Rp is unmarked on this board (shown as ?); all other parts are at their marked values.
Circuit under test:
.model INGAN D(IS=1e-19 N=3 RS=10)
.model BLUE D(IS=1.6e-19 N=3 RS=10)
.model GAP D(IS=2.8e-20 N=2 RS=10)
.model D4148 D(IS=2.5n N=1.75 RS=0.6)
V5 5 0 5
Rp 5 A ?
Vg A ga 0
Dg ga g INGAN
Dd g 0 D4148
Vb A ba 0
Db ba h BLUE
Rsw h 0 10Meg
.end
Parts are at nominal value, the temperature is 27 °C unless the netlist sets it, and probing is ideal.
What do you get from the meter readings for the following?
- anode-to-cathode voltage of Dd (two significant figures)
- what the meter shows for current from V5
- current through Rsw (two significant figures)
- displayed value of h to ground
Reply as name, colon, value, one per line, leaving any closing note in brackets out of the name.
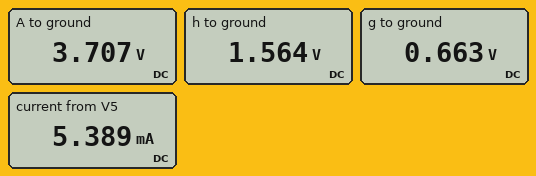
anode-to-cathode voltage of Dd: 660 mV
what the meter shows for current from V5: 5.389 mA
current through Rsw: 160 nA
displayed value of h to ground: 1.564 V
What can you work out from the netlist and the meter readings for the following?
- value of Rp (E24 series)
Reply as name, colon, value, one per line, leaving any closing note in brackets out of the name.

value of Rp: 240 Ω
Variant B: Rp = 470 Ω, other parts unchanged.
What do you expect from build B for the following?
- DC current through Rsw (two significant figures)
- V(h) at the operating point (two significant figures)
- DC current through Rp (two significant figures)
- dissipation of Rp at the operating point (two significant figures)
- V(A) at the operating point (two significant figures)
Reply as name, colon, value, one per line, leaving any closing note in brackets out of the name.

DC current through Rsw: 150 nA
V(h) at the operating point: 1.5 V
DC current through Rp: 3.0 mA
dissipation of Rp at the operating point: 4.1 mW
V(A) at the operating point: 3.6 V
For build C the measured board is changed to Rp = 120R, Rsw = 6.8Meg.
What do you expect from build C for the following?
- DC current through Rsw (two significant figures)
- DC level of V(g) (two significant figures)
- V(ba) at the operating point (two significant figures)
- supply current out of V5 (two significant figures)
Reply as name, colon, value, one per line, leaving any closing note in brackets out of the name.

DC current through Rsw: 240 nA
DC level of V(g): 690 mV
V(ba) at the operating point: 3.8 V
supply current out of V5: 9.8 mA
